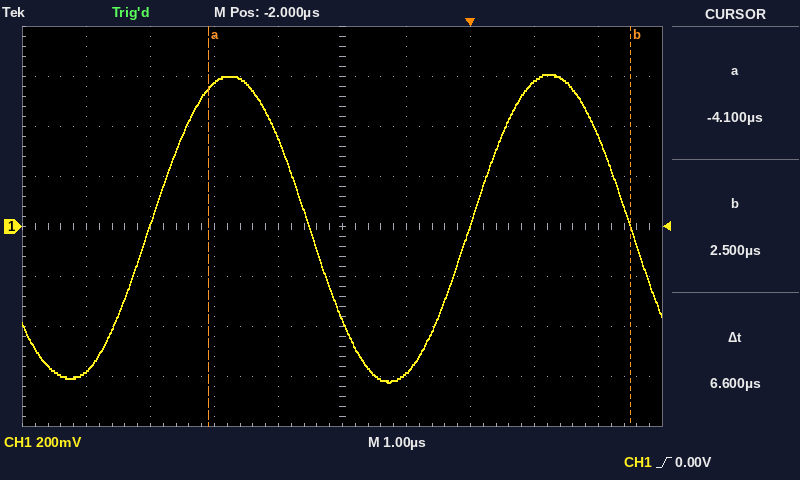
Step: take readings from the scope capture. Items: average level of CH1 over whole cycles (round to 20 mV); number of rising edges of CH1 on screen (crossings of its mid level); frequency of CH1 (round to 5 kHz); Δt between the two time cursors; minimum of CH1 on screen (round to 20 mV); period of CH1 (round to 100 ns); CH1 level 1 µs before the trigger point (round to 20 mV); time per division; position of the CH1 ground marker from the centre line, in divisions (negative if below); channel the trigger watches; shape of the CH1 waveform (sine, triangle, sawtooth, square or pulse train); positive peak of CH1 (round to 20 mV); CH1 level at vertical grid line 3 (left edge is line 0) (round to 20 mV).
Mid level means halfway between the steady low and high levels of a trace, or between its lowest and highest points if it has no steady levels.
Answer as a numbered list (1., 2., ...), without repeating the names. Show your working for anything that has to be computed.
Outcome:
1. (600 mV + (-620 mV)) / 2 ≈ 0 mV
2. 2
3. 1 / 5.0 µs ≈ 200 kHz
4. 6.6 µs
5. -620 mV
6. 5.0 µs
7. -580 mV
8. 1 µs
9. 0.0 div
10. CH1
11. sine
12. 600 mV
13. 580 mV
